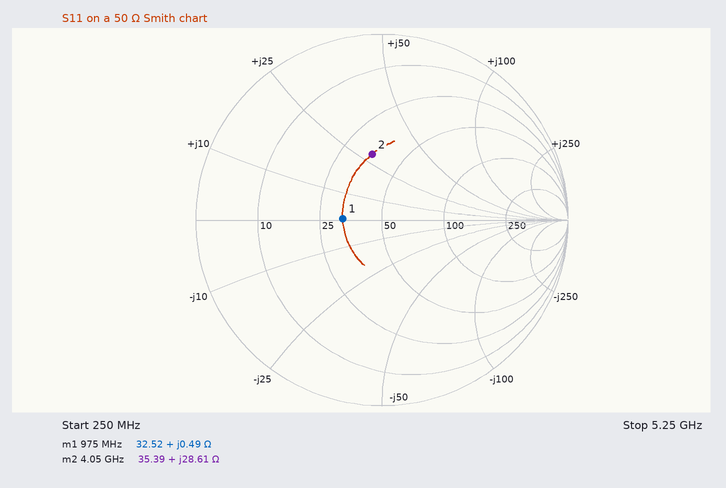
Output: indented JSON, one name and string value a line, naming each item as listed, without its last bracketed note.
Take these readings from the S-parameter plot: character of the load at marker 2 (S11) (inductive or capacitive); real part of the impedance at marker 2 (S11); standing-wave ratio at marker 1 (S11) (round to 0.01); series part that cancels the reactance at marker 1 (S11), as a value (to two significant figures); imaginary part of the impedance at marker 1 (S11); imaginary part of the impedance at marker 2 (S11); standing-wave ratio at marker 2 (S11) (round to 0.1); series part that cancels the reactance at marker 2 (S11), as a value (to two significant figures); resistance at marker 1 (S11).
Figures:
{
  "character of the load at marker 2 (S11)": "inductive",
  "real part of the impedance at marker 2": "35.39 Ω",
  "standing-wave ratio at marker 1 (S11)": "1.54",
  "series part that cancels the reactance at marker 1 (S11), as a value": "330 pF",
  "imaginary part of the impedance at marker 1": "+0.49 Ω",
  "imaginary part of the impedance at marker 2": "+28.61 Ω",
  "standing-wave ratio at marker 2 (S11)": "2.1",
  "series part that cancels the reactance at marker 2 (S11), as a value": "1.4 pF",
  "resistance at marker 1": "32.52 Ω"
}
